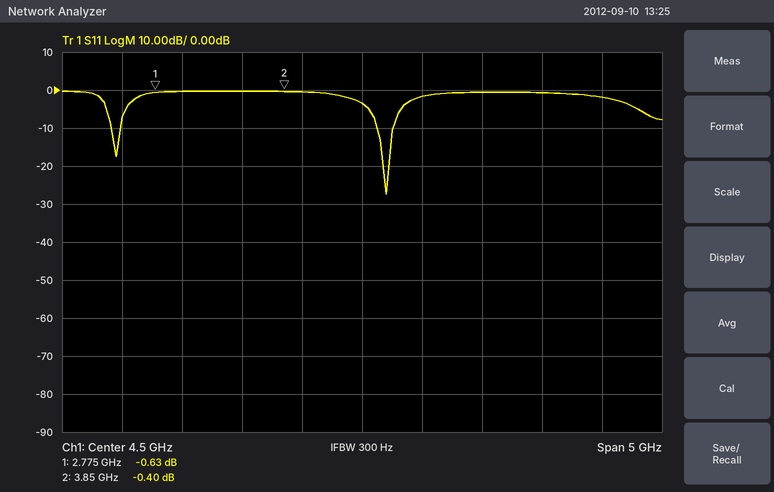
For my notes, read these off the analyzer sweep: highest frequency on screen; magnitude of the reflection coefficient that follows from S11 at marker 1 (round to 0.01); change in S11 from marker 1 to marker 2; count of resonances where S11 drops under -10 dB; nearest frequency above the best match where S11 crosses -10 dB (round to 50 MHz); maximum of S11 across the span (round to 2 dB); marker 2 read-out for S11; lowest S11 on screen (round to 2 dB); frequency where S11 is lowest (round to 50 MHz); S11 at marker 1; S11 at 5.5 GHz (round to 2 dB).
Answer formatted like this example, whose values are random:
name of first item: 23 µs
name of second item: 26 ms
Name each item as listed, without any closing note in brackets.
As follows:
highest frequency on screen: 7 GHz
magnitude of the reflection coefficient that follows from S11 at marker 1: 0.93
change in S11 from marker 1 to marker 2: 0.23 dB
count of resonances where S11 drops under -10 dB: 2
nearest frequency above the best match where S11 crosses -10 dB: 4.75 GHz
maximum of S11 across the span: 0 dB
marker 2 read-out for S11: -0.40 dB
lowest S11 on screen: -28 dB
frequency where S11 is lowest: 4.70 GHz
S11 at marker 1: -0.63 dB
S11 at 5.5 GHz: 0 dB
